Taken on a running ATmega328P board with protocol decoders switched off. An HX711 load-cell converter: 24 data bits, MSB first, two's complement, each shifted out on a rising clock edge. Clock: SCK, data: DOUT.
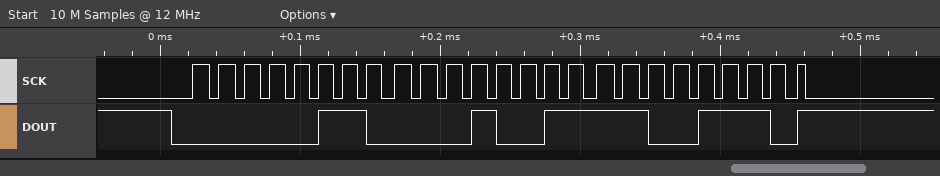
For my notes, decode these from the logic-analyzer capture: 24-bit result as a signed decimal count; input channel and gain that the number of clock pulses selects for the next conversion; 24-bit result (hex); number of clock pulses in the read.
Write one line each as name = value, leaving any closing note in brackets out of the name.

24-bit result as a signed decimal count = 398286
input channel and gain that the number of clock pulses selects for the next conversion = channel A, gain 128
24-bit result = 0x0613CE
number of clock pulses in the read = 25
